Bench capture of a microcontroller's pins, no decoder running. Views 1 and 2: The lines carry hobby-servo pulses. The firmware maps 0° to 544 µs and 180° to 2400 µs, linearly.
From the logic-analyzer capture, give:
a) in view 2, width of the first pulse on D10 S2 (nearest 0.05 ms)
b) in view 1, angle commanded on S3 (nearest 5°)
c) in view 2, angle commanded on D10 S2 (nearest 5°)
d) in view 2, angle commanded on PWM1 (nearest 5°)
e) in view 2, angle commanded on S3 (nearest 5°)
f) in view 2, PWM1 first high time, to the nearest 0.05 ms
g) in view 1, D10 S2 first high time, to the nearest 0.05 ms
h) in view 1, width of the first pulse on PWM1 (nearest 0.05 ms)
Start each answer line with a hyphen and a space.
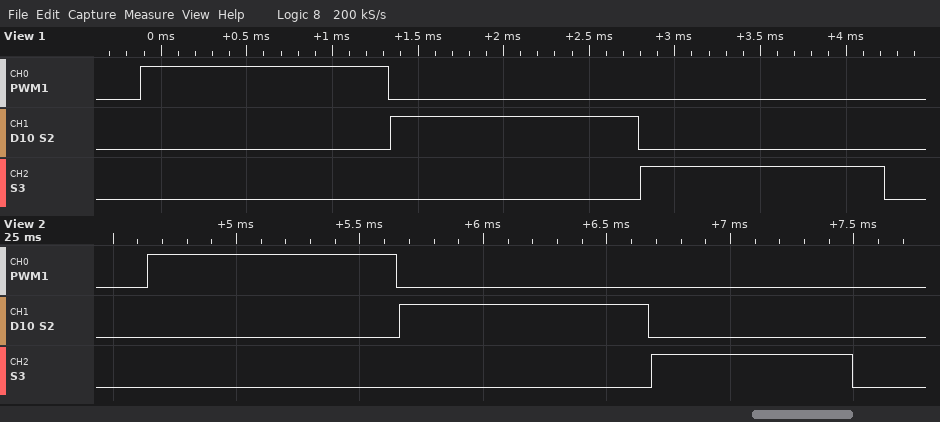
- 1.00 ms
- 85°
- 45°
- 45°
- 25°
- 1.00 ms
- 1.45 ms
- 1.45 ms
